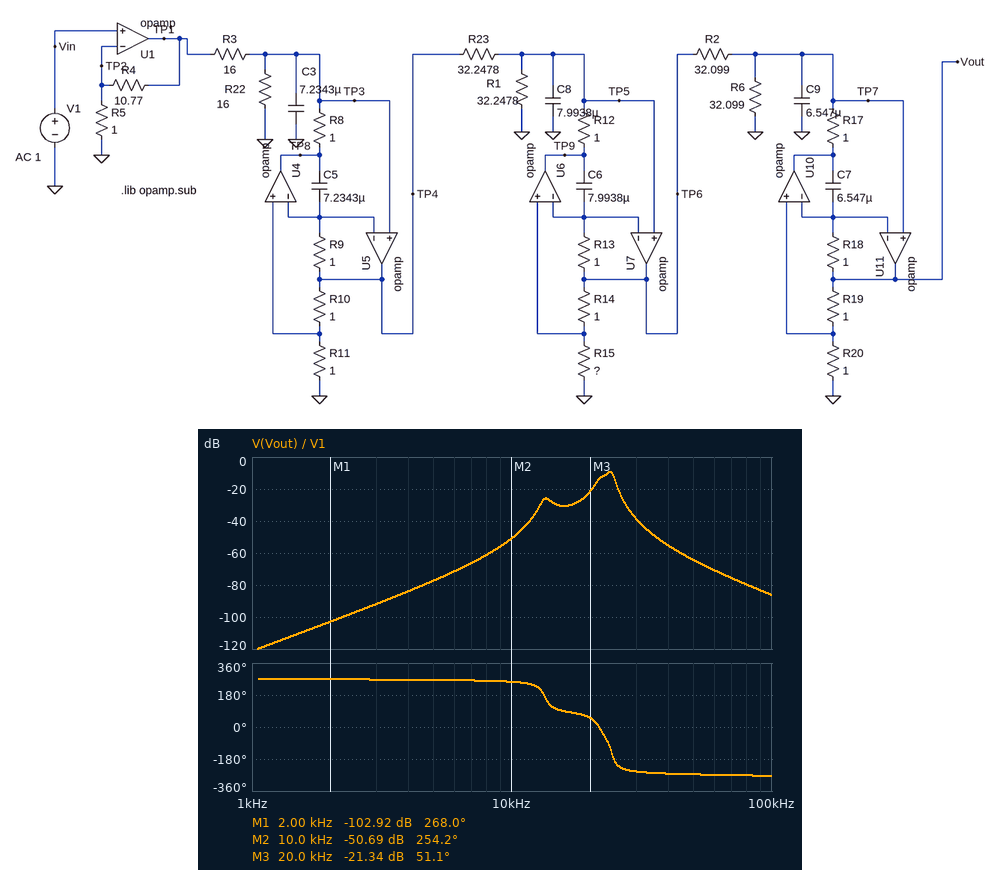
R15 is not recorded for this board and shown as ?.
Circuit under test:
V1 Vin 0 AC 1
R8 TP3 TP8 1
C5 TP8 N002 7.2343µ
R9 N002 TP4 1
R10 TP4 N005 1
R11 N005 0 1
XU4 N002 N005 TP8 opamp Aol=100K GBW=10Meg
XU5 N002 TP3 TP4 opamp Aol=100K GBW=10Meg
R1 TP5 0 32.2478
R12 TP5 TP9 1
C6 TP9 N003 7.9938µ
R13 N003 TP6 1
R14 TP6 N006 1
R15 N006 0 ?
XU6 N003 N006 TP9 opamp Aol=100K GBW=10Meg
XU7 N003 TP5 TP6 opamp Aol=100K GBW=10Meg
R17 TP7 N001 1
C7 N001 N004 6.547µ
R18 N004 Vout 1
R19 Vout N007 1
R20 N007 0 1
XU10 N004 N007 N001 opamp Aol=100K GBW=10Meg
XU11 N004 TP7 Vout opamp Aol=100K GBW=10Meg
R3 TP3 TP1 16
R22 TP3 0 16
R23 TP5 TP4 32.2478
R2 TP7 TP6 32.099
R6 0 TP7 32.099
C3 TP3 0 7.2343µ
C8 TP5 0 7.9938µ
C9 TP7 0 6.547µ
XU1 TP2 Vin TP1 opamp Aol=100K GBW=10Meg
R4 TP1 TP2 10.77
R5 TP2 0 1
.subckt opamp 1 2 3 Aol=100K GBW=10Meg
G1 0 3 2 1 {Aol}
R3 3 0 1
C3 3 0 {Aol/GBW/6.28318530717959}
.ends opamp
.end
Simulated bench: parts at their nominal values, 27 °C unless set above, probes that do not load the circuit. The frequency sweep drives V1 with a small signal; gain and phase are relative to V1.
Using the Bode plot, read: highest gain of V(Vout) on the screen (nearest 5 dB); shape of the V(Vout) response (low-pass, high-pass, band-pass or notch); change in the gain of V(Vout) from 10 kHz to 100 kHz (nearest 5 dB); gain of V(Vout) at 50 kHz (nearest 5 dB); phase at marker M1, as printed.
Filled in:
-10 dB
band-pass
-35 dB
-65 dB
268.0 deg
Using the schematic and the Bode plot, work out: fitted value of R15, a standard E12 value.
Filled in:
2.2 Ω
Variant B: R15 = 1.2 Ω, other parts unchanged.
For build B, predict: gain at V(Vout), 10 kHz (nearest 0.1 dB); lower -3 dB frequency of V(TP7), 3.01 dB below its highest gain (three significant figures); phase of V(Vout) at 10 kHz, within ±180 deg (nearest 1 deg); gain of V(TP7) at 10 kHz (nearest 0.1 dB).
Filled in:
-57.8 dB
21.4 kHz
-100 deg
-63.8 dB
